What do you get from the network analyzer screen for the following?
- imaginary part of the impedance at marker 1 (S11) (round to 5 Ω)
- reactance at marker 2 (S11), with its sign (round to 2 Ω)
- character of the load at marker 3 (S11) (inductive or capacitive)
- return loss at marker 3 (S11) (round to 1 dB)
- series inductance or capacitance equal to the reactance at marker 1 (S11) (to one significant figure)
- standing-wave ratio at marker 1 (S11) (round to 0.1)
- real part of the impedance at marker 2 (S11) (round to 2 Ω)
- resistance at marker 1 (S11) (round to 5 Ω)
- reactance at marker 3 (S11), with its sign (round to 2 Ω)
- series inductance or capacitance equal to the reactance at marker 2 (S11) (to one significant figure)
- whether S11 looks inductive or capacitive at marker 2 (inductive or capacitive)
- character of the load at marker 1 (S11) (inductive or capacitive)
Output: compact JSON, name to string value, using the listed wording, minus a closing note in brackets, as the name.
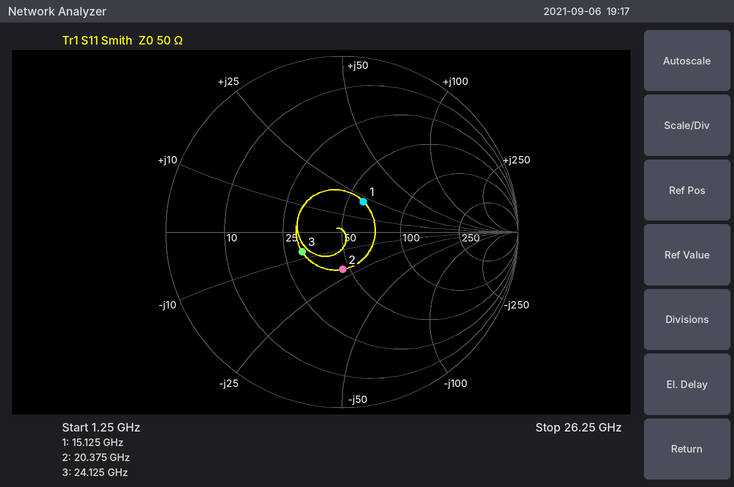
{"imaginary part of the impedance at marker 1 (S11)": "+20 Ω", "reactance at marker 2 (S11), with its sign": "-20 Ω", "character of the load at marker 3 (S11)": "capacitive", "return loss at marker 3 (S11)": "12 dB", "series inductance or capacitance equal to the reactance at marker 1 (S11)": "200 pH", "standing-wave ratio at marker 1 (S11)": "1.5", "real part of the impedance at marker 2 (S11)": "46 Ω", "resistance at marker 1 (S11)": "60 Ω", "reactance at marker 3 (S11), with its sign": "-8 Ω", "series inductance or capacitance equal to the reactance at marker 2 (S11)": "400 fF", "whether S11 looks inductive or capacitive at marker 2": "capacitive", "character of the load at marker 1 (S11)": "inductive"}
